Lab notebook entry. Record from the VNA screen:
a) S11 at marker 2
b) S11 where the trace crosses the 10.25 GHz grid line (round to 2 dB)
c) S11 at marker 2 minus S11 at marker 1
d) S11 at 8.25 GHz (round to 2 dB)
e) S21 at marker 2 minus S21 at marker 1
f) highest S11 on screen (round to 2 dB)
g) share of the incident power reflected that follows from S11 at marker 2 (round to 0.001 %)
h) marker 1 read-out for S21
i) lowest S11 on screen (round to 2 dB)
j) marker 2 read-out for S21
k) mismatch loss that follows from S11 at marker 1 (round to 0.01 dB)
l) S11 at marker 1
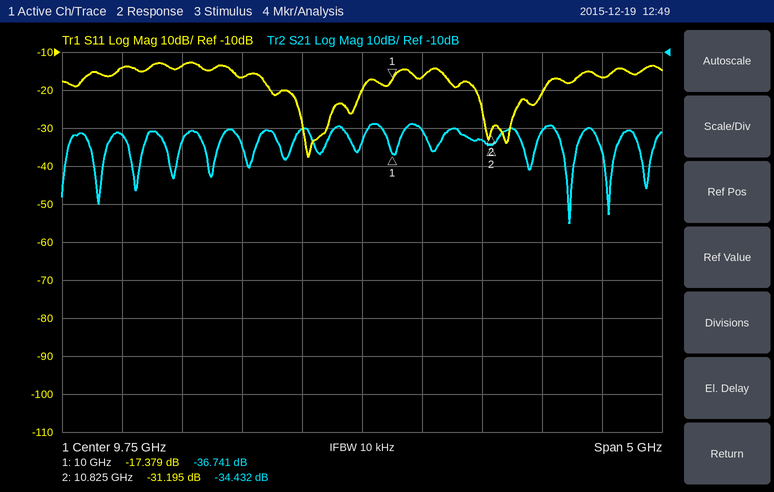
-31.195 dB
-16 dB
-13.816 dB
-14 dB
2.309 dB
-12 dB
0.076 %
-36.741 dB
-38 dB
-34.432 dB
0.08 dB
-17.379 dB
